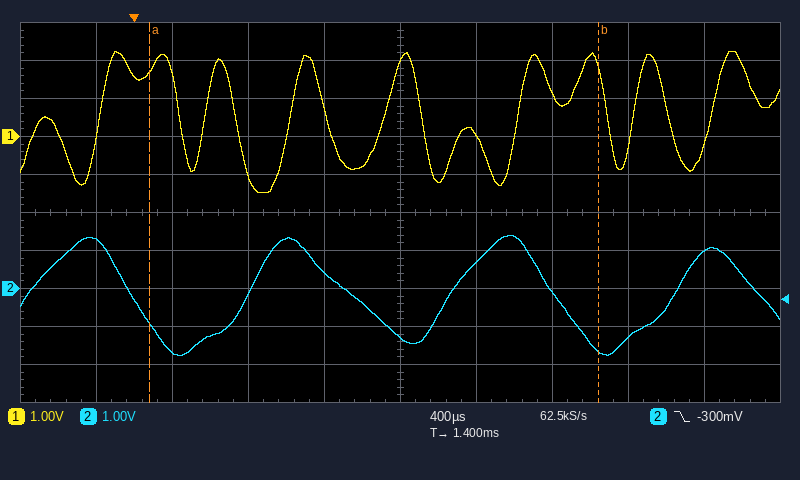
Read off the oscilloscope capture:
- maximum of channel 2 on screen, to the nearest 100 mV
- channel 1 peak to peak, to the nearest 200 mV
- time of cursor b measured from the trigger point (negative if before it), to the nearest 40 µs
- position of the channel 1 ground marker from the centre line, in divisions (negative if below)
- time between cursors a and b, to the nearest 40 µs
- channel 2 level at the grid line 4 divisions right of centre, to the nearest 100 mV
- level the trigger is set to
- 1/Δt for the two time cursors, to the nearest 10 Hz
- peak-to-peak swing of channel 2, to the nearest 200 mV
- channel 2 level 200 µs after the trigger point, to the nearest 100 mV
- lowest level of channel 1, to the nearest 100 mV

1.4 V
3.8 V
+2.44 ms
+2.0 div
2.36 ms
1.0 V
-300 mV
420 Hz
3.2 V
-1.7 V
-1.5 V
